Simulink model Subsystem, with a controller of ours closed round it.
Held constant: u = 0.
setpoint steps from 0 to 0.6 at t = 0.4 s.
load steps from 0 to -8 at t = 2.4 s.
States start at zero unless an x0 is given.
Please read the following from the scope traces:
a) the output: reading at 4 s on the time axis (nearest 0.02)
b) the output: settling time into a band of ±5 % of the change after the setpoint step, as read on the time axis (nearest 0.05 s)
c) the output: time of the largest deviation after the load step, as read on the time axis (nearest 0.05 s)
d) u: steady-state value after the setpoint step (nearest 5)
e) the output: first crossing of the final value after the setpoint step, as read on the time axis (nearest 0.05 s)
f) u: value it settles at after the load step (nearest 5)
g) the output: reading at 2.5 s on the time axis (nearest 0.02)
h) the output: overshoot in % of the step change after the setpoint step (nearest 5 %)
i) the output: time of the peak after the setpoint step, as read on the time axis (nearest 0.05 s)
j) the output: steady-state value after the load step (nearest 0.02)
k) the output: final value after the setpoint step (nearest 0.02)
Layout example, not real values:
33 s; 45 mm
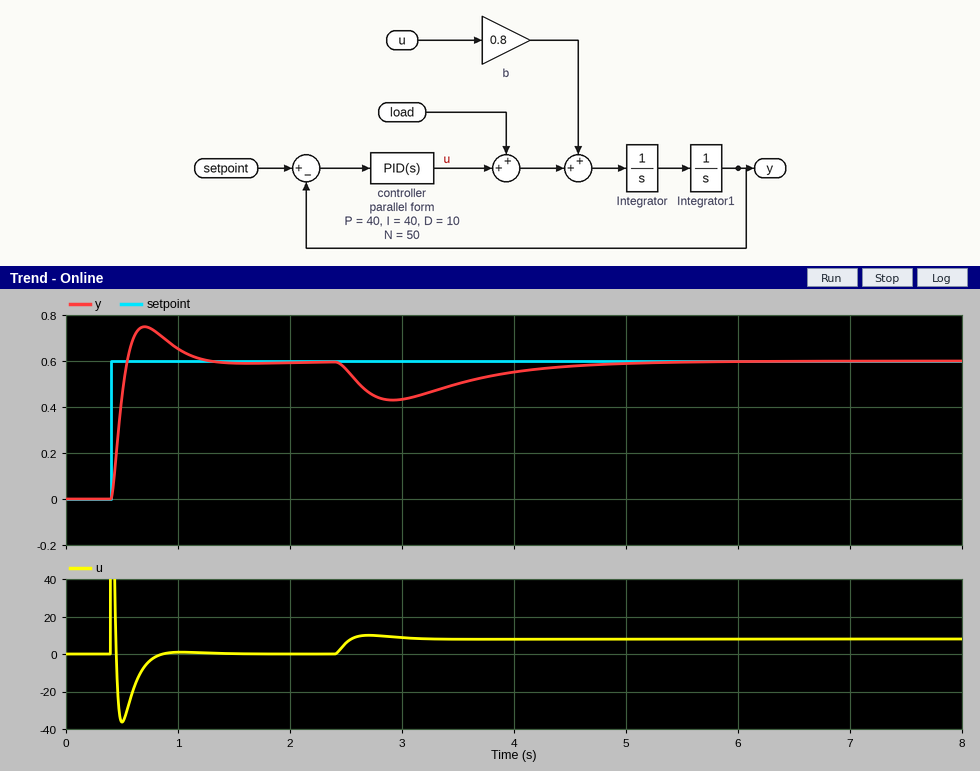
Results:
0.56; 1.10 s; 2.90 s; 0; 0.55 s; 10; 0.56; 25 %; 0.70 s; 0.60; 0.60
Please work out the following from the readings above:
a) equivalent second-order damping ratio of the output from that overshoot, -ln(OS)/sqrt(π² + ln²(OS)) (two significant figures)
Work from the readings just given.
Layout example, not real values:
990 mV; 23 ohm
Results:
0.40
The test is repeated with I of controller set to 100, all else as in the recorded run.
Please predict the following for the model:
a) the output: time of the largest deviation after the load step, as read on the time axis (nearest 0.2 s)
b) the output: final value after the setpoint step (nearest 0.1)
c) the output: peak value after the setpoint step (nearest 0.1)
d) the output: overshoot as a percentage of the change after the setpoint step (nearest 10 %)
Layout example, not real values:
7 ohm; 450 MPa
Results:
2.8 s; 0.6; 0.8; 30 %
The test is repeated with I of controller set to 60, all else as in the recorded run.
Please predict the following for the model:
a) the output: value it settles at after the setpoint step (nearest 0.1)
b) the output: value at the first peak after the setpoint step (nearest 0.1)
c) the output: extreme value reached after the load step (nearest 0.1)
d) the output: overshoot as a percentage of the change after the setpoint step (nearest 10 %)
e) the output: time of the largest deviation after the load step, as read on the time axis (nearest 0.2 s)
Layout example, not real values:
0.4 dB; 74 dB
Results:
0.6; 0.8; 0.4; 30 %; 2.8 s
